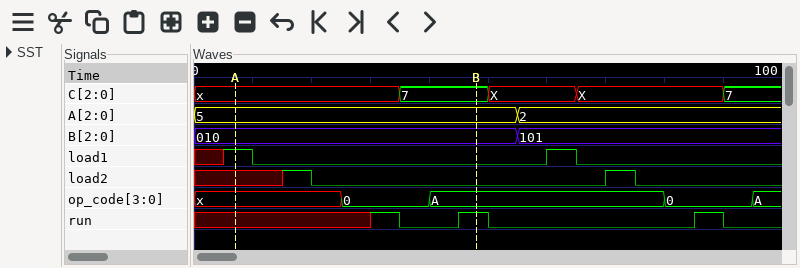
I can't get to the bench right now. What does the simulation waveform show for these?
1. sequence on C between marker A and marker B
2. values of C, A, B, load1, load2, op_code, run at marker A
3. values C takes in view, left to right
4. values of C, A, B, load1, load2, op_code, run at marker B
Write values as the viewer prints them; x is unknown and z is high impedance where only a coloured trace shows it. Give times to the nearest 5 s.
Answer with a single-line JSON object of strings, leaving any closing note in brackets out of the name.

{"sequence on C between marker A and marker B": "x, 7", "values of C, A, B, load1, load2, op_code, run at marker A": "C=x, A=5, B=010, load1=1, load2=x, op_code=x, run=x", "values C takes in view, left to right": "x, 7, X, X, 7", "values of C, A, B, load1, load2, op_code, run at marker B": "C=7, A=5, B=010, load1=0, load2=0, op_code=A, run=1"}
